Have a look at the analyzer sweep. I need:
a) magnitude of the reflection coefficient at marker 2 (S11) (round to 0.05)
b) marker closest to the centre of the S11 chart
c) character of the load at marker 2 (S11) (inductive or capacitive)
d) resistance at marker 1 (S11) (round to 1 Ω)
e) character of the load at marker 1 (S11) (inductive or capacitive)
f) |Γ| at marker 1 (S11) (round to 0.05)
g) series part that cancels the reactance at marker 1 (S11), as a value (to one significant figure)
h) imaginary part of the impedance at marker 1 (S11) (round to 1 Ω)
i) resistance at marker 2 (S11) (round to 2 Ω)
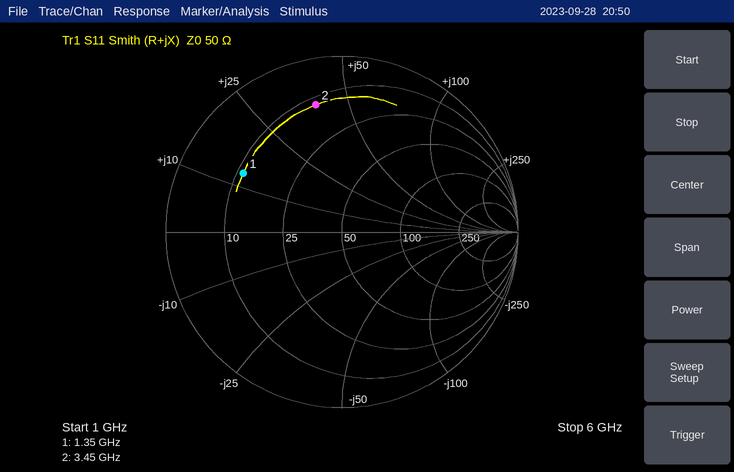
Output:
0.75
marker 1
inductive
11 Ω
inductive
0.65
9 pF
+13 Ω
12 Ω
